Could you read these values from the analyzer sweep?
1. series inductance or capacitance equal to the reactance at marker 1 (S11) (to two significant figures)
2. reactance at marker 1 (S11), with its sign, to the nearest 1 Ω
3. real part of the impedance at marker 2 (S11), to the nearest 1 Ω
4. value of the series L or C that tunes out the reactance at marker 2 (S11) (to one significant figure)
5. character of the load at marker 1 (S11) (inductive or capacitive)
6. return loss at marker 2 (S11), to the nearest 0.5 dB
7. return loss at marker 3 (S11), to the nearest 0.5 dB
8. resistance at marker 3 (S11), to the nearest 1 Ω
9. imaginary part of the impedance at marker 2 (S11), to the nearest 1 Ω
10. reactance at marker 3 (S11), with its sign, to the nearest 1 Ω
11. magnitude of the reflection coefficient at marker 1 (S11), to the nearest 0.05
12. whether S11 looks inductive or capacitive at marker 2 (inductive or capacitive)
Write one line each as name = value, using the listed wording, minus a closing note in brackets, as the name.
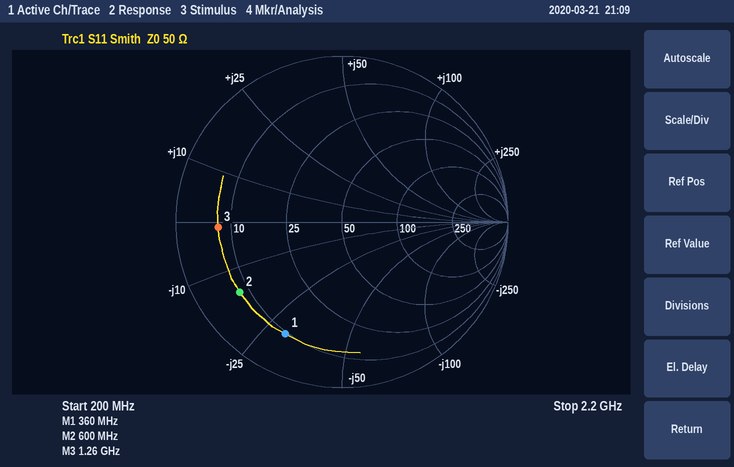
series inductance or capacitance equal to the reactance at marker 1 (S11) = 15 pF
reactance at marker 1 (S11), with its sign, to the nearest 1 Ω = -30 Ω
real part of the impedance at marker 2 (S11), to the nearest 1 Ω = 8 Ω
value of the series L or C that tunes out the reactance at marker 2 (S11) = 4 nH
character of the load at marker 1 (S11) = capacitive
return loss at marker 2 (S11), to the nearest 0.5 dB = 2.5 dB
return loss at marker 3 (S11), to the nearest 0.5 dB = 2.5 dB
resistance at marker 3 (S11), to the nearest 1 Ω = 7 Ω
imaginary part of the impedance at marker 2 (S11), to the nearest 1 Ω = -15 Ω
reactance at marker 3 (S11), with its sign, to the nearest 1 Ω = -1 Ω
magnitude of the reflection coefficient at marker 1 (S11), to the nearest 0.05 = 0.75
whether S11 looks inductive or capacitive at marker 2 = capacitive
